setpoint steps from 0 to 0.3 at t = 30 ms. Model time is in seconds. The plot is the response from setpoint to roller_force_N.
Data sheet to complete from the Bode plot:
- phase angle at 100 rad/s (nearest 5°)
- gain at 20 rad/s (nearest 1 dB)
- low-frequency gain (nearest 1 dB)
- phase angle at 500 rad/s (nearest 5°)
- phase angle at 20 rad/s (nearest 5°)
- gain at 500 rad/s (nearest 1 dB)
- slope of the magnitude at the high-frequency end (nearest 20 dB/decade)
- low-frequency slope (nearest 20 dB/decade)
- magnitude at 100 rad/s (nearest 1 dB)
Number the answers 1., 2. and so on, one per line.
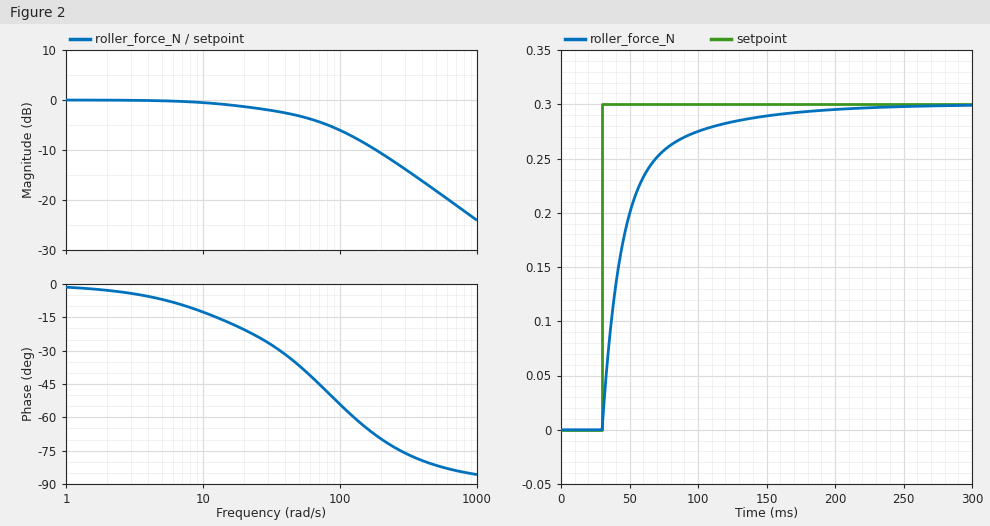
1. -55°
2. -1 dB
3. 0 dB
4. -80°
5. -20°
6. -18 dB
7. -20 dB/decade
8. 0 dB/decade
9. -6 dB
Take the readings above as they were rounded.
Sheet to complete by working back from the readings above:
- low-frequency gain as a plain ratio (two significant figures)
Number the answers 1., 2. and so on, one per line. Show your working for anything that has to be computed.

1. 10^(0 / 20) = 1.0
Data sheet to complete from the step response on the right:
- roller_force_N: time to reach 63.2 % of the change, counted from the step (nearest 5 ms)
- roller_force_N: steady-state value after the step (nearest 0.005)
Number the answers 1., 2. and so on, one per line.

1. 20 ms
2. 0.300
